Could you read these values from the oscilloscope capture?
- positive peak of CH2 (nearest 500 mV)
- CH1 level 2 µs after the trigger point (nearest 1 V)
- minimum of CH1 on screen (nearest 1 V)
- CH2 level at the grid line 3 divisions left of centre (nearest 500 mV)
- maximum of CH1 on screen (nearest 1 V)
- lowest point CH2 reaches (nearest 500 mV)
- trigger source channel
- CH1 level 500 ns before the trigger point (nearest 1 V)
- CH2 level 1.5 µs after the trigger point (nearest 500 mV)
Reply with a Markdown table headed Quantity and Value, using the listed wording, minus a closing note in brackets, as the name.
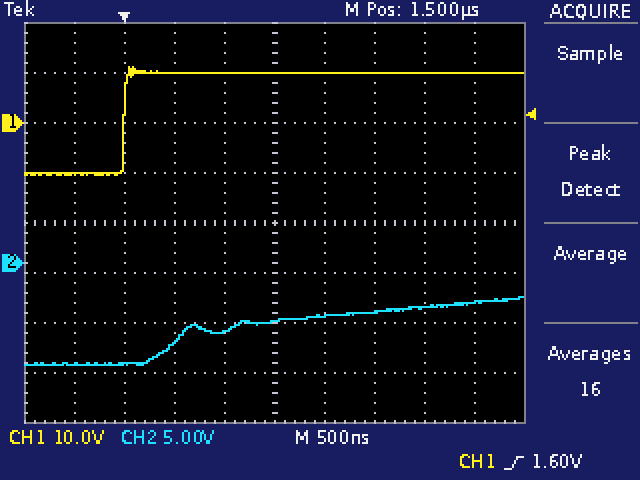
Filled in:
| Quantity | Value |
|---|---|
| positive peak of CH2 | -3.5 V |
| CH1 level 2 µs after the trigger point | 10 V |
| minimum of CH1 on screen | -10 V |
| CH2 level at the grid line 3 divisions left of centre | -10.0 V |
| maximum of CH1 on screen | 11 V |
| lowest point CH2 reaches | -10.0 V |
| trigger source channel | CH1 |
| CH1 level 500 ns before the trigger point | -10 V |
| CH2 level 1.5 µs after the trigger point | -6.0 V |
